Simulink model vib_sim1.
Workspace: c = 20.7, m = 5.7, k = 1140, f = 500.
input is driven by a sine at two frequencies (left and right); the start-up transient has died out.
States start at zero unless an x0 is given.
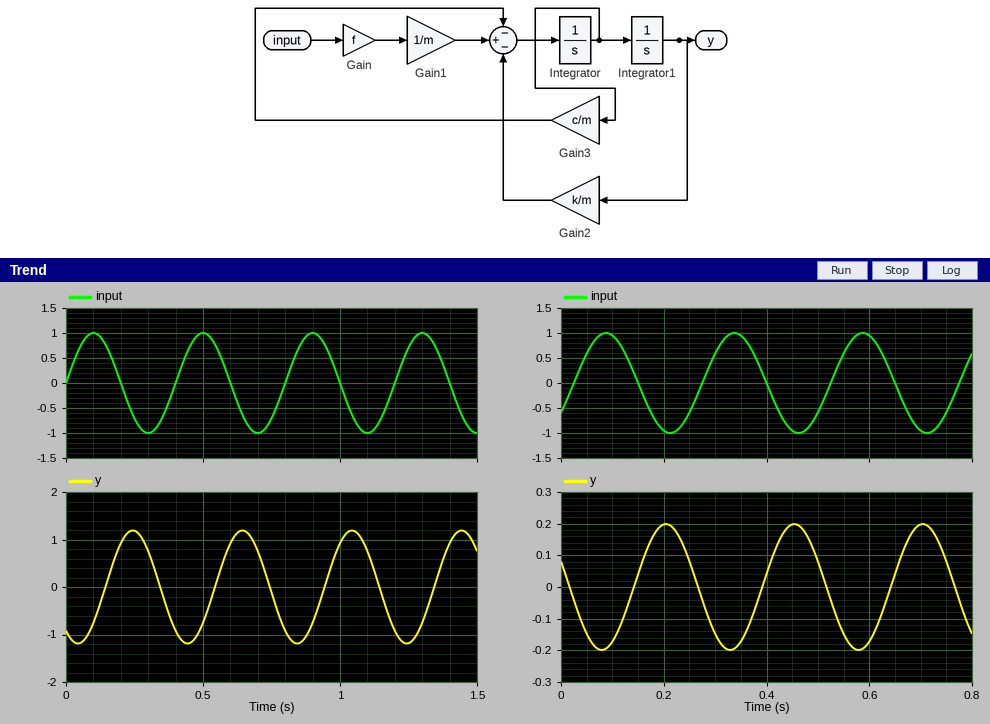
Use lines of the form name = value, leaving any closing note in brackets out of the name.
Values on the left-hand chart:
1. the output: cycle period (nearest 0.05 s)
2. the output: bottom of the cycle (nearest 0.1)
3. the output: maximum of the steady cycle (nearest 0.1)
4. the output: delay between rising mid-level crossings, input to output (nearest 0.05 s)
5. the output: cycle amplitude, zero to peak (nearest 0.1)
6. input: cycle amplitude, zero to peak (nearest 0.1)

the output: cycle period = 0.40 s
the output: bottom of the cycle = -1.2
the output: maximum of the steady cycle = 1.2
the output: delay between rising mid-level crossings, input to output = 0.15 s
the output: cycle amplitude, zero to peak = 1.2
input: cycle amplitude, zero to peak = 1.0
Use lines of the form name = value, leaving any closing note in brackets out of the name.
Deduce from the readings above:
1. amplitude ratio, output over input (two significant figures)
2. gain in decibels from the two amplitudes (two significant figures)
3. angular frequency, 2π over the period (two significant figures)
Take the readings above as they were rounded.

amplitude ratio, output over input = 1.2
gain in decibels from the two amplitudes = 1.6 dB
angular frequency, 2π over the period = 16 rad/s
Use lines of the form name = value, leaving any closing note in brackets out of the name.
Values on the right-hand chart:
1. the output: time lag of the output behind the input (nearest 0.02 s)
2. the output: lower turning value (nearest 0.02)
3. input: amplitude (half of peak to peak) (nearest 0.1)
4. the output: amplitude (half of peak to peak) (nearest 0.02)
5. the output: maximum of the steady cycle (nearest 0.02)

the output: time lag of the output behind the input = 0.12 s
the output: lower turning value = -0.20
input: amplitude (half of peak to peak) = 1.0
the output: amplitude (half of peak to peak) = 0.20
the output: maximum of the steady cycle = 0.20
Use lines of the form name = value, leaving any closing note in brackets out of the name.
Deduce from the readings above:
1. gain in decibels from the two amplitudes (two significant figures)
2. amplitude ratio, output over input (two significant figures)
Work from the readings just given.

gain in decibels from the two amplitudes = -14 dB
amplitude ratio, output over input = 0.20
